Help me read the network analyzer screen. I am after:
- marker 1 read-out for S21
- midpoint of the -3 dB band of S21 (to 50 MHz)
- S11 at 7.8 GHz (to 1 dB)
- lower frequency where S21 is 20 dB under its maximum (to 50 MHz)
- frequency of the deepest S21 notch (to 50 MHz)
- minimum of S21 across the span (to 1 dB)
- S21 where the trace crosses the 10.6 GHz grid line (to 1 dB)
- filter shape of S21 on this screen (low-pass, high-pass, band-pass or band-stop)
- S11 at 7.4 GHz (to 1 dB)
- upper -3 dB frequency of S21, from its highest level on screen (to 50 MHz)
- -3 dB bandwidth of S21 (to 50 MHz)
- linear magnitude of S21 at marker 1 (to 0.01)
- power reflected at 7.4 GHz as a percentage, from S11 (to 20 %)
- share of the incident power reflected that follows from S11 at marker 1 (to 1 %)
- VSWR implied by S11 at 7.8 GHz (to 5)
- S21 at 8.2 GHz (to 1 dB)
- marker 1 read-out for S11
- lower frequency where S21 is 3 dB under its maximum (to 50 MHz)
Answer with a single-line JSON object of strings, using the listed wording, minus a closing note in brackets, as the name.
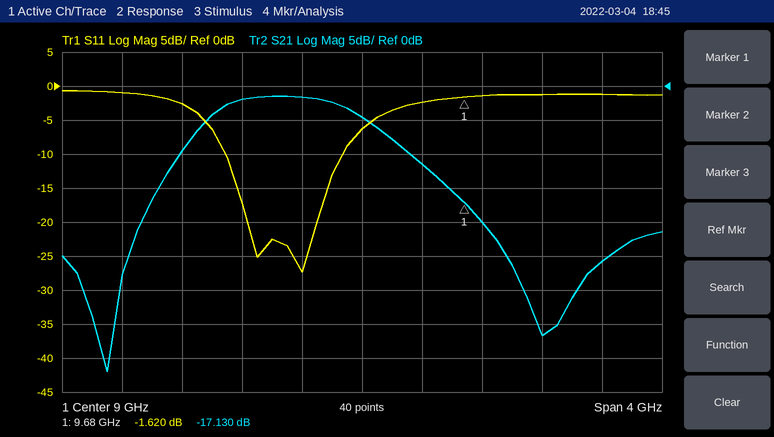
{"marker 1 read-out for S21": "-17.130 dB", "midpoint of the -3 dB band of S21": "8.50 GHz", "S11 at 7.8 GHz": "-3 dB", "lower frequency where S21 is 20 dB under its maximum": "7.50 GHz", "frequency of the deepest S21 notch": "7.30 GHz", "minimum of S21 across the span": "-42 dB", "S21 where the trace crosses the 10.6 GHz grid line": "-26 dB", "filter shape of S21 on this screen": "band-pass", "S11 at 7.4 GHz": "-1 dB", "upper -3 dB frequency of S21, from its highest level on screen": "9.00 GHz", "-3 dB bandwidth of S21": "1.00 GHz", "linear magnitude of S21 at marker 1": "0.14", "power reflected at 7.4 GHz as a percentage, from S11": "80 %", "share of the incident power reflected that follows from S11 at marker 1": "69 %", "VSWR implied by S11 at 7.8 GHz": "5", "S21 at 8.2 GHz": "-2 dB", "marker 1 read-out for S11": "-1.620 dB", "lower frequency where S21 is 3 dB under its maximum": "8.00 GHz"}
